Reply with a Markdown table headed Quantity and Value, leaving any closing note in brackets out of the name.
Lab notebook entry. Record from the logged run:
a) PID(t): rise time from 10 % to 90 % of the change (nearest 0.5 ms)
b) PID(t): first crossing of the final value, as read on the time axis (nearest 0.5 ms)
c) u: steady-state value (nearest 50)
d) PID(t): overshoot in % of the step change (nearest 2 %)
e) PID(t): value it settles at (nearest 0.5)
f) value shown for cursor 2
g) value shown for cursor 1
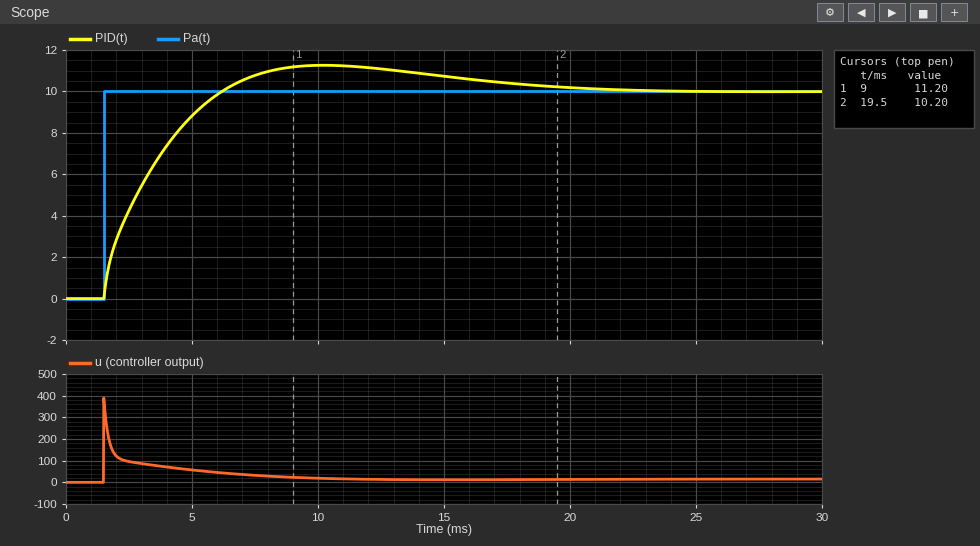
| Quantity | Value |
|---|---|
| PID(t): rise time from 10 % to 90 % of the change | 3.5 ms |
| PID(t): first crossing of the final value, as read on the time axis | 6.0 ms |
| u: steady-state value | 0 |
| PID(t): overshoot in % of the step change | 12 % |
| PID(t): value it settles at | 10.0 |
| value shown for cursor 2 | 10.20 |
| value shown for cursor 1 | 11.20 |
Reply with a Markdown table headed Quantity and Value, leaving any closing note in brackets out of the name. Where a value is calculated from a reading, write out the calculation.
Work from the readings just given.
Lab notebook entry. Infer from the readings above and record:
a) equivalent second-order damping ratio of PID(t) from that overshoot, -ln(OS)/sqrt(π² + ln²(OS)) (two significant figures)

| Quantity | Value |
|---|---|
| equivalent second-order damping ratio of PID(t) from that overshoot, -ln(OS)/sqrt(π² + ln²(OS)) | ln(0.12) = -2.120; 2.120 / sqrt(9.870 + 4.496) = 0.56 |
